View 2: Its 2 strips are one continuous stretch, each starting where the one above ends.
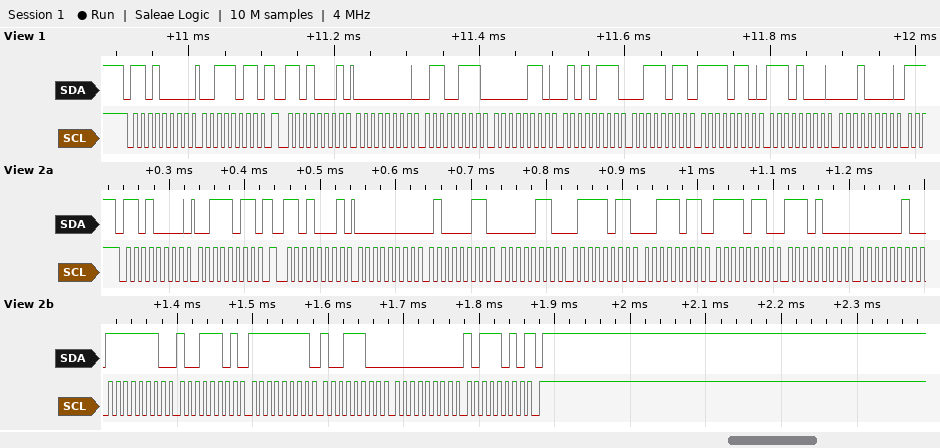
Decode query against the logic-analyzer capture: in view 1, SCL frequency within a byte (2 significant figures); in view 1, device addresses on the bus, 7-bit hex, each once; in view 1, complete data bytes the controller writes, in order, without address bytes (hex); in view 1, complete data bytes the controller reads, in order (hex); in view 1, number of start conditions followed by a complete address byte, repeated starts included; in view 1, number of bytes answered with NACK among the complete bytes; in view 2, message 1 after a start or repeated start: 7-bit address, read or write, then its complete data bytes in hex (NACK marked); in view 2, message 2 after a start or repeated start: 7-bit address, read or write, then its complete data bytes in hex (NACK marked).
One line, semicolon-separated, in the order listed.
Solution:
100 kHz; 0x68; 3B; 00 67 06 57 3B F6 E8 10; 2; 0; 0x68 write: 3B; 0x68 read: 00 43 06 7B 3B F6 E8 02 FE 9D FF 9C 00 BA NACK
